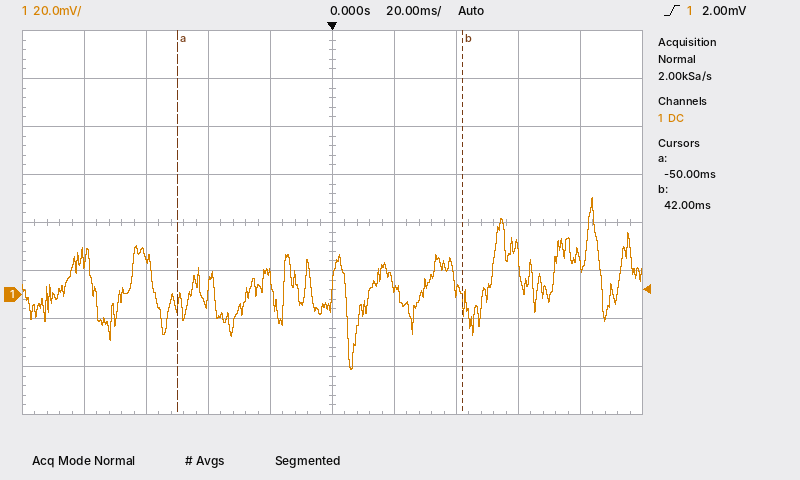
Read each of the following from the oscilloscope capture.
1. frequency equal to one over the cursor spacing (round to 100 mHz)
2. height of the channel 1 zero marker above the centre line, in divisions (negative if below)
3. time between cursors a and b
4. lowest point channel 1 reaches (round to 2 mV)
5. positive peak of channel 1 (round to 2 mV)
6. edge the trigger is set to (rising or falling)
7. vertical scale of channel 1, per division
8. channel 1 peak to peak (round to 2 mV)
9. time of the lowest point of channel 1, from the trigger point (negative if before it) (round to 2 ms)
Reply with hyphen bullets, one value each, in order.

- 10.9 Hz
- -1.5 div
- 92 ms
- -32 mV
- 40 mV
- rising
- 20 mV
- 72 mV
- +6 ms
